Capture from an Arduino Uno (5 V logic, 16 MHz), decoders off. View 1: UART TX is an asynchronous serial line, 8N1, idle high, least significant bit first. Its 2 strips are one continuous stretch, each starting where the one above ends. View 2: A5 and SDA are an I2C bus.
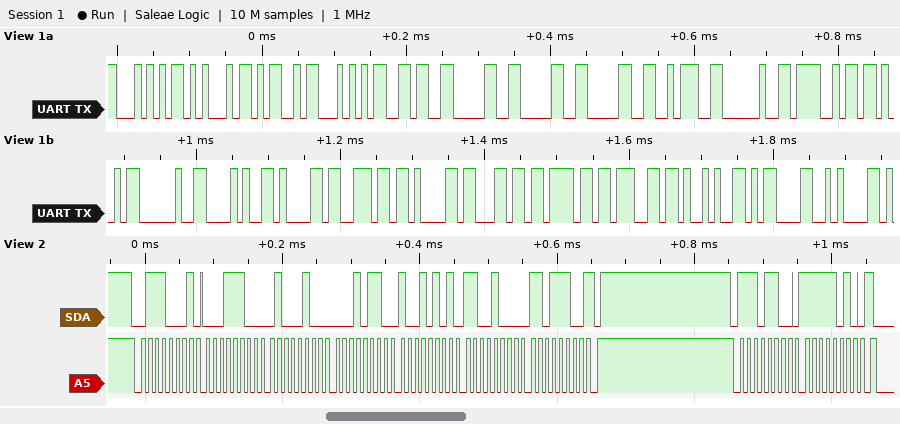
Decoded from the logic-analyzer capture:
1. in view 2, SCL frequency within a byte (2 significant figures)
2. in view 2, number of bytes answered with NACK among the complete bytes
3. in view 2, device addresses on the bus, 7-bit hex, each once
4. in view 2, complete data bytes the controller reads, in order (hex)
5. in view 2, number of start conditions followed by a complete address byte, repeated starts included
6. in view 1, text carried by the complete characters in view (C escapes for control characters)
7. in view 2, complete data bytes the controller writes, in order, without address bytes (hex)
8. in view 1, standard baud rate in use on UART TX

100 kHz
1
0x38 0x76
1C 44 16 95 C8 DC
2
"TEMT6000: OK (analog)\r\n"
FA
115200 baud
